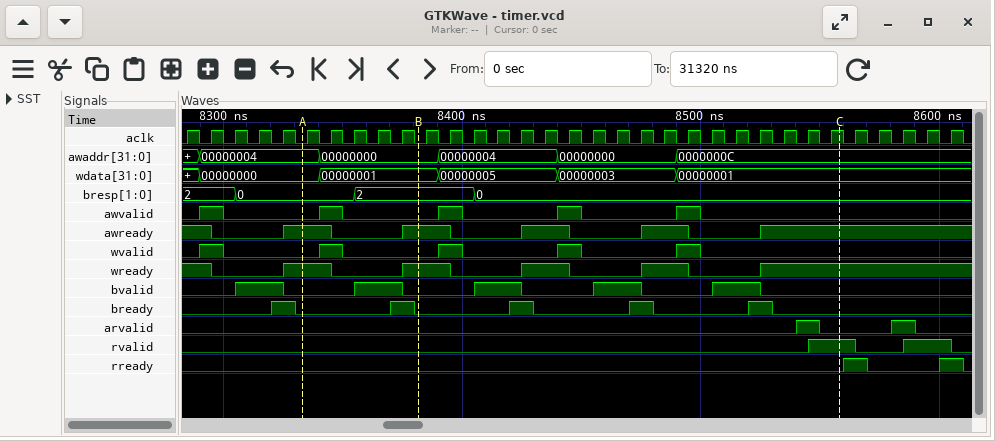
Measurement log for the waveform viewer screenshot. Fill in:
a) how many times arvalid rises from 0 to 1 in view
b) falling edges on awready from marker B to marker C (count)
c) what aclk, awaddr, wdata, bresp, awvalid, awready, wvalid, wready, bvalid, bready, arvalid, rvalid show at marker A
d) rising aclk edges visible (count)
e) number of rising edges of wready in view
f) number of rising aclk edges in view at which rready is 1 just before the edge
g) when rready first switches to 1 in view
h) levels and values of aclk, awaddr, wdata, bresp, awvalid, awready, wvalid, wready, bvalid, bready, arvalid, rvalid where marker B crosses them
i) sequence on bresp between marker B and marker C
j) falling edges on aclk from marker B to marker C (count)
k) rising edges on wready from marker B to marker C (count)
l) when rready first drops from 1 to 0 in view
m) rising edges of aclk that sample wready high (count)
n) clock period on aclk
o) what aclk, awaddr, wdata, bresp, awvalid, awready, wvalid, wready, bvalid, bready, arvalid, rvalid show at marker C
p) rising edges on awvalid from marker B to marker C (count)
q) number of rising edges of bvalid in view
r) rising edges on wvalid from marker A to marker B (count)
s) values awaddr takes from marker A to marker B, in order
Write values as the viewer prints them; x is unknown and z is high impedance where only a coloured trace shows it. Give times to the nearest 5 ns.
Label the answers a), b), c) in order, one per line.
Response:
a) 2
b) 3
c) aclk=0, awaddr=00000004, wdata=00000000, bresp=0, awvalid=0, awready=1, wvalid=0, wready=1, bvalid=0, bready=0, arvalid=0, rvalid=0
d) 33
e) 5
f) 2
g) 8560 ns
h) aclk=0, awaddr=00000000, wdata=00000001, bresp=2, awvalid=0, awready=1, wvalid=0, wready=1, bvalid=0, bready=0, arvalid=0, rvalid=0
i) 2, 0
j) 17
k) 3
l) 8570 ns
m) 18
n) 10 ns
o) aclk=1, awaddr=0000000C, wdata=00000001, bresp=0, awvalid=0, awready=1, wvalid=0, wready=1, bvalid=0, bready=0, arvalid=0, rvalid=1
p) 3
q) 5
r) 1
s) 00000004, 00000000
